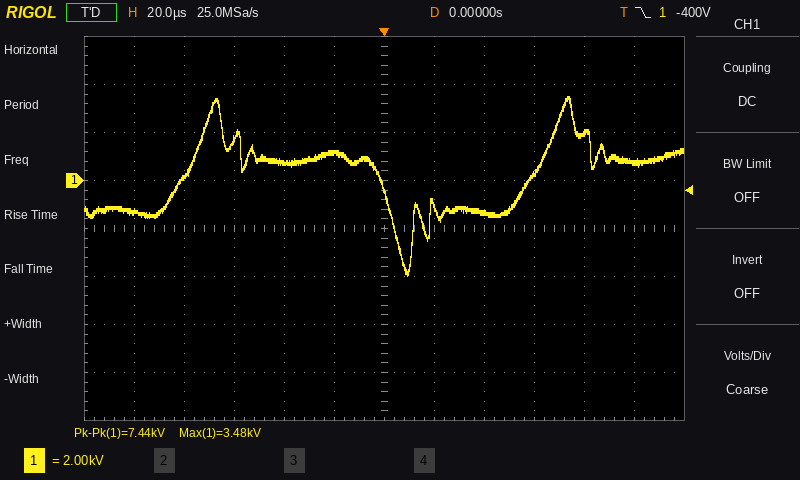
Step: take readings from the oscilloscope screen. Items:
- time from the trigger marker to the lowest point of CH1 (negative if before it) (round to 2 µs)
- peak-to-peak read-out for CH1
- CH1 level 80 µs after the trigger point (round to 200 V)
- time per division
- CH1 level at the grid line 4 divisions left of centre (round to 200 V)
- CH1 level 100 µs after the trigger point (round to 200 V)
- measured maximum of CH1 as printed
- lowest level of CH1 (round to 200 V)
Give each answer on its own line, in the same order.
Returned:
+10 µs
7.44 kV
2.0 kV
20 µs
200 V
800 V
3.48 kV
-4.0 kV
